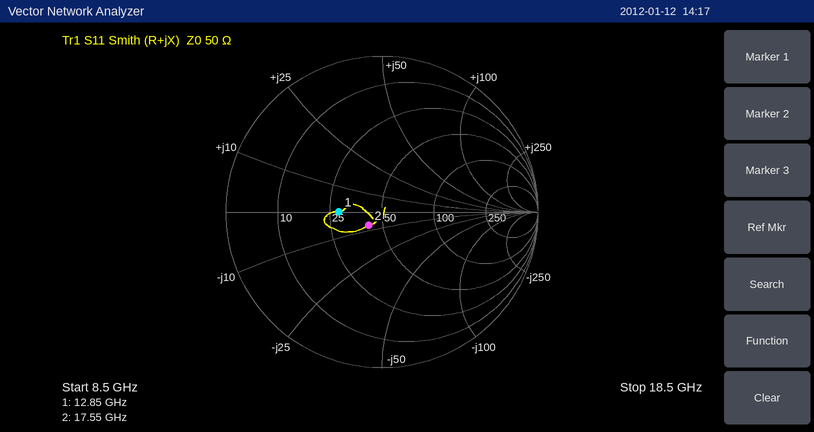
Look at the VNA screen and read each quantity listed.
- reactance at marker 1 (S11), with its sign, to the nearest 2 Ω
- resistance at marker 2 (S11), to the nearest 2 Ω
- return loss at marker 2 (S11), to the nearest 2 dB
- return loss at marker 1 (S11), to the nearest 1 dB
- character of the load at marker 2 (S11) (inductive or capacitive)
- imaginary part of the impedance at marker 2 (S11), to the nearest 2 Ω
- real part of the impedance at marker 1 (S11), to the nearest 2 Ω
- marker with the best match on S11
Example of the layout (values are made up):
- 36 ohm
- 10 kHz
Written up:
- 0 Ω
- 42 Ω
- 18 dB
- 11 dB
- capacitive
- -8 Ω
- 28 Ω
- marker 2
